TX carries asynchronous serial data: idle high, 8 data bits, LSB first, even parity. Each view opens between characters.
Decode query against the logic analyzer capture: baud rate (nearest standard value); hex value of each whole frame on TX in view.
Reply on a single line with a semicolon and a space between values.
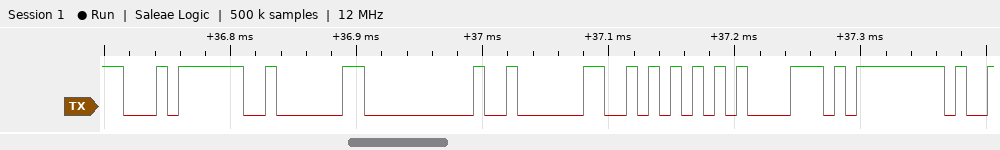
115200 baud; F4, 02, 00, 02, AA, E1, FF
